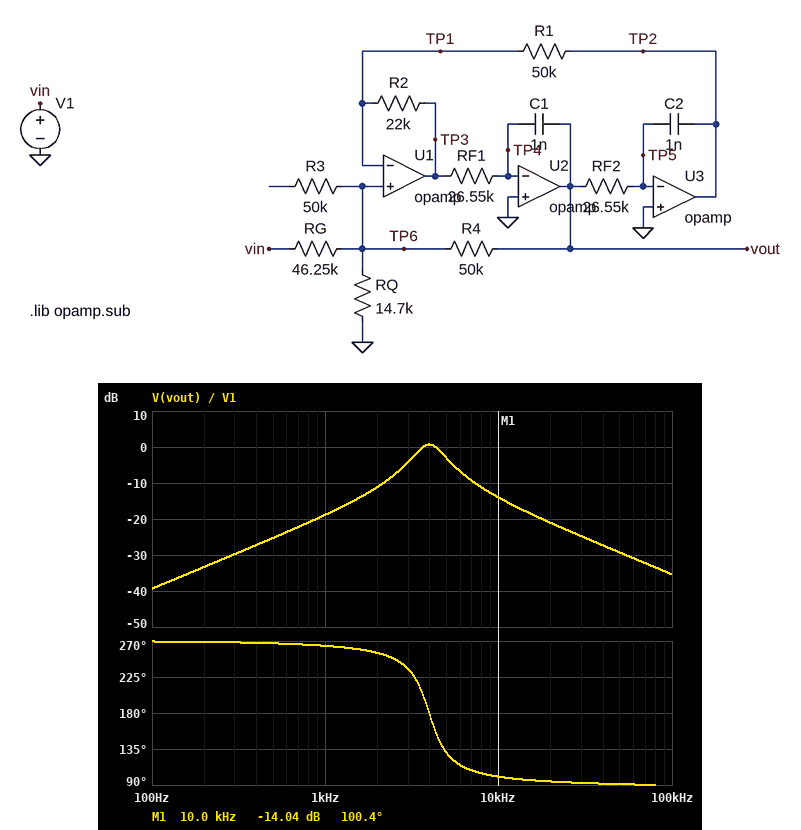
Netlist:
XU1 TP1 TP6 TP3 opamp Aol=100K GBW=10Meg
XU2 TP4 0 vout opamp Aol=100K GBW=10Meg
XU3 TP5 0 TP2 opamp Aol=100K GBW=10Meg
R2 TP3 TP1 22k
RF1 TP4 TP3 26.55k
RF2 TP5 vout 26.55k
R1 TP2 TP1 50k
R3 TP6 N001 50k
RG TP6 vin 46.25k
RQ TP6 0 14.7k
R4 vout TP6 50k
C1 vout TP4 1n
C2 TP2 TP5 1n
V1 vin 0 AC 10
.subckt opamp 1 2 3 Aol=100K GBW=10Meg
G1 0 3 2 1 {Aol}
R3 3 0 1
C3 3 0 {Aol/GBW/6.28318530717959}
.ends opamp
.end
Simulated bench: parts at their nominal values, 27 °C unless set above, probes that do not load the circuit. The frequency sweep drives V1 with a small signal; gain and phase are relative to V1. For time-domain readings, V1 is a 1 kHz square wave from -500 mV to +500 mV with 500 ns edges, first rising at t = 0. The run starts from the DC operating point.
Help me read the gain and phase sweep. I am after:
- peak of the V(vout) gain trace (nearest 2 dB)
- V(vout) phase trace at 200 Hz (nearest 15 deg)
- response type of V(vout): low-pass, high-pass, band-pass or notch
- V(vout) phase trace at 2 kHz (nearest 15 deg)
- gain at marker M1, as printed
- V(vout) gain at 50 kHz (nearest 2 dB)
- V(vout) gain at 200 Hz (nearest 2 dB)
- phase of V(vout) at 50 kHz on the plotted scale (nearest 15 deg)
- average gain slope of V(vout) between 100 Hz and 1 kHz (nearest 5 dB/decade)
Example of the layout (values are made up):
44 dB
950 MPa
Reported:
0 dB
270 deg
band-pass
255 deg
-14.04 dB
-30 dB
-34 dB
90 deg
20 dB/decade
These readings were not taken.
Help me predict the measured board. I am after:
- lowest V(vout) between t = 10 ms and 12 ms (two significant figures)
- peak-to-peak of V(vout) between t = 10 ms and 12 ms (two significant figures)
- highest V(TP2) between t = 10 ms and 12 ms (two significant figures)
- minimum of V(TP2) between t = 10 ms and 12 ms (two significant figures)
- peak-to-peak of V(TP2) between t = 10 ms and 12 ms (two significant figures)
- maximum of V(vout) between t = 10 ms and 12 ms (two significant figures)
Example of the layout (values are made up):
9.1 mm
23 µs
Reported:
-300 mV
600 mV
640 mV
-640 mV
1.3 V
300 mV
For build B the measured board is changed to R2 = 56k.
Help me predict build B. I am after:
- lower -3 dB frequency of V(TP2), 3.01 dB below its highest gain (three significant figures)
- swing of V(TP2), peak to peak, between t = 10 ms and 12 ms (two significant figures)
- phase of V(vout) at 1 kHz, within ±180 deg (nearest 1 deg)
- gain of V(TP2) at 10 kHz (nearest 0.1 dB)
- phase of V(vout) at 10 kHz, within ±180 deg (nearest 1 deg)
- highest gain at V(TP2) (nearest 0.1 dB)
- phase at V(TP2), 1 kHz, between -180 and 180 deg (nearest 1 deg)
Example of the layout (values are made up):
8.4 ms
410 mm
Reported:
4.82 kHz
780 mV
-93 deg
-12.6 dB
111 deg
0.4 dB
-3 deg
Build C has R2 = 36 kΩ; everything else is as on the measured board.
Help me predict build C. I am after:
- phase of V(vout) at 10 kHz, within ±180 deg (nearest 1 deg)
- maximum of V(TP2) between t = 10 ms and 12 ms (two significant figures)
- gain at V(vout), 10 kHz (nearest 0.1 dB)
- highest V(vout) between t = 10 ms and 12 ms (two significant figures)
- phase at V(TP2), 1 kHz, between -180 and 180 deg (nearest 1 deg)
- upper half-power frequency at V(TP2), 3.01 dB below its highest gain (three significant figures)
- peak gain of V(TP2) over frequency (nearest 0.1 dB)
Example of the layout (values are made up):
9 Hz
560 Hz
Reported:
104 deg
510 mV
-11.5 dB
330 mV
-4 deg
5.78 kHz
2.3 dB
